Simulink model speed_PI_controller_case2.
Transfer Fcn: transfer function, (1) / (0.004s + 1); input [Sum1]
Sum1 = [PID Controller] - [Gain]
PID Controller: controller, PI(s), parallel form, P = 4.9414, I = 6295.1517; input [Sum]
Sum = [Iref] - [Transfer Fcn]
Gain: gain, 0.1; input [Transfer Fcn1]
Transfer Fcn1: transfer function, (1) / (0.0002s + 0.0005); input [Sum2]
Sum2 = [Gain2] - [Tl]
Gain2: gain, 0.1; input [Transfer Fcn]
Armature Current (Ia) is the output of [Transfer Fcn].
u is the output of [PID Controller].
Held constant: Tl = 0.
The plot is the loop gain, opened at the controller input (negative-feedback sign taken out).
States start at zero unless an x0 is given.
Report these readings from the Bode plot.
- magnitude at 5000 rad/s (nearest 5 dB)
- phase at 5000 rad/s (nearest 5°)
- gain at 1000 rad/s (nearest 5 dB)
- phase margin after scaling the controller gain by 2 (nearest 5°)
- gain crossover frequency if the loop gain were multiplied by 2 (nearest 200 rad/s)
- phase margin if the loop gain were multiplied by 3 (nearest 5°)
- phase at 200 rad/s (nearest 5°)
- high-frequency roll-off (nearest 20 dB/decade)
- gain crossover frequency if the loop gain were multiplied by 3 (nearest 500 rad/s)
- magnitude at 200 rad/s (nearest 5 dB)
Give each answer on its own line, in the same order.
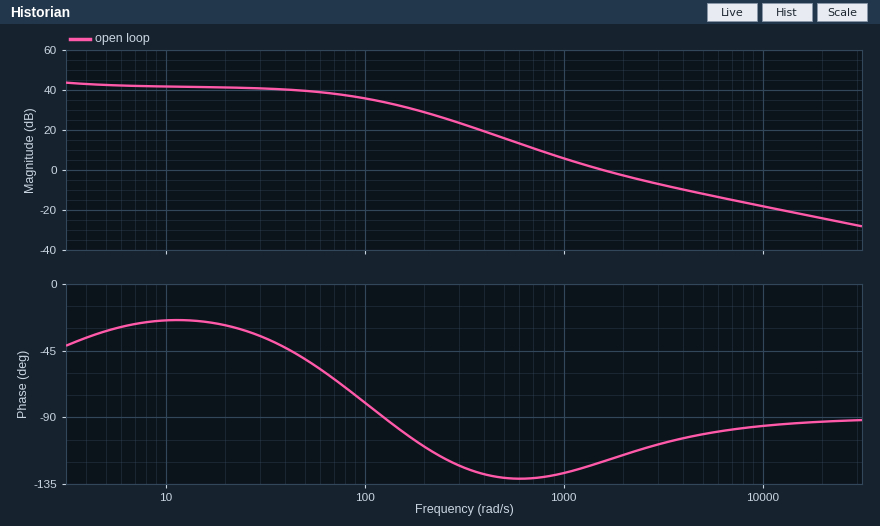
-10 dB
-100°
5 dB
70°
2800 rad/s
75°
-110°
-20 dB/decade
4000 rad/s
30 dB
